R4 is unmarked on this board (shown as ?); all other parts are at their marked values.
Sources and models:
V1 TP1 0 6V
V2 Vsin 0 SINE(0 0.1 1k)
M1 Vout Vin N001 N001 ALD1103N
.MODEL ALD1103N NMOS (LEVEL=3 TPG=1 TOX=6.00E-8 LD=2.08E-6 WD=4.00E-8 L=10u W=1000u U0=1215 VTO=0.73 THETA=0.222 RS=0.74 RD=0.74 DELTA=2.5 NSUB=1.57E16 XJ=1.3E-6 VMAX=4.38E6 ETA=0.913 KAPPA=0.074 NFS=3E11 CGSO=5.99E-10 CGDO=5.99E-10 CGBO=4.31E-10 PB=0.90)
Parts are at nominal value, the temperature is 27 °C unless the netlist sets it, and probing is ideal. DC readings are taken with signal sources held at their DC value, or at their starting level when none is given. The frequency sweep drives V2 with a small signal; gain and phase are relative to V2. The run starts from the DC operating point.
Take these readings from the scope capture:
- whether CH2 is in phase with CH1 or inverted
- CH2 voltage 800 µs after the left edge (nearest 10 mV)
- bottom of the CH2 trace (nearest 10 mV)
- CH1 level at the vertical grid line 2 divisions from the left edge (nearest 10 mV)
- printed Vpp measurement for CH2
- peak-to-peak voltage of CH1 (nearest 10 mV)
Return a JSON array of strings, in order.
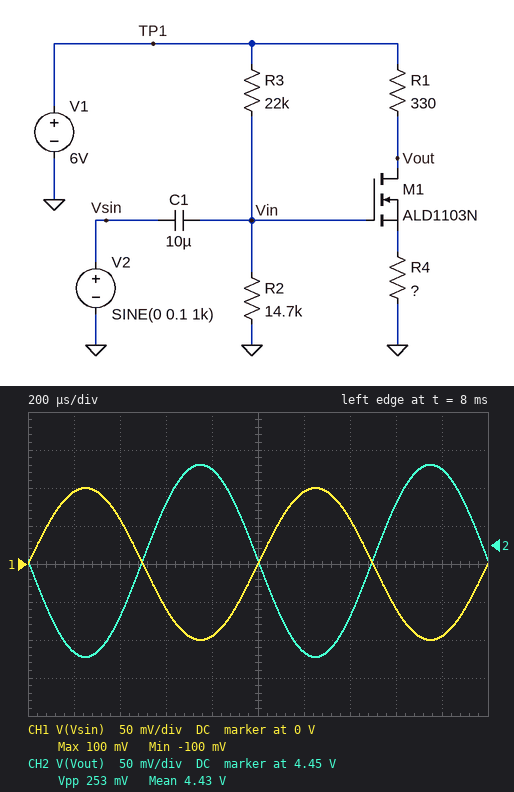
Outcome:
["inverted", "4.55 V", "4.30 V", "60 mV", "253 mV", "200 mV"]
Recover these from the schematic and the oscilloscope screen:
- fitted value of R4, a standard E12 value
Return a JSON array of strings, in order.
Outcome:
["120 Ω"]
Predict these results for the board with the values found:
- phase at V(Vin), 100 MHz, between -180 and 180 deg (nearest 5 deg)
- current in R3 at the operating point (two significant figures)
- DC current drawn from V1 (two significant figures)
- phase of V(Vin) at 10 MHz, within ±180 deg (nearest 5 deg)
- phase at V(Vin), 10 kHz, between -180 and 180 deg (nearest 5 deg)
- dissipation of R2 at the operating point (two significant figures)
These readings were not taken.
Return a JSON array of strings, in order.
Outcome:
["0 deg", "160 µA", "4.9 mA", "0 deg", "0 deg", "390 µW"]
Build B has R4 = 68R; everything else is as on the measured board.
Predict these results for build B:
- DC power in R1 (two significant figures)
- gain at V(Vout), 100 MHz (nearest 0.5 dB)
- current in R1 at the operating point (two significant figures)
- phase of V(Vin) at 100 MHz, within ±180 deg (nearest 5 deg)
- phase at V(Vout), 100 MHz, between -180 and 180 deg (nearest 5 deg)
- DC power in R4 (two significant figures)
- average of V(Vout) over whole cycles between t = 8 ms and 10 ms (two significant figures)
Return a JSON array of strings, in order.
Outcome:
["12 mW", "4.5 dB", "6.0 mA", "0 deg", "165 deg", "2.4 mW", "4.0 V"]
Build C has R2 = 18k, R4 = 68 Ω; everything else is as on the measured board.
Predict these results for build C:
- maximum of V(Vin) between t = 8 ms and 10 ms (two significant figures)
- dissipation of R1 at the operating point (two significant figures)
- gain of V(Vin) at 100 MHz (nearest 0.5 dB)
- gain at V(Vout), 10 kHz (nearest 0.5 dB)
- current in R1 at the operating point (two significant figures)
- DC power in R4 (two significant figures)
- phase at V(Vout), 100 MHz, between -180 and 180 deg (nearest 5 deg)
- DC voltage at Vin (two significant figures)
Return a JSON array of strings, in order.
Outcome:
["2.8 V", "19 mW", "0 dB", "5.0 dB", "7.5 mA", "3.9 mW", "165 deg", "2.7 V"]
